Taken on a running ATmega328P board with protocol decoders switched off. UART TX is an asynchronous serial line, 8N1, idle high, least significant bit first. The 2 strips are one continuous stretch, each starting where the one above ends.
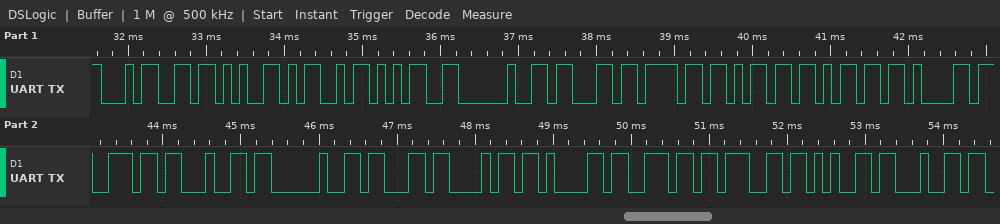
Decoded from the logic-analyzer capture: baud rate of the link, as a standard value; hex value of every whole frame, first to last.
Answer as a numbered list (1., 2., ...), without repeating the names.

1. 9600 baud
2. 0x34 0x2B 0x4D 0x35 0x20 0x63 0x6F 0x6D 0x6D 0x61 0x6E 0x64 0x20 0x63 0x68 0x61 0x6E 0x67 0x65 0x64
